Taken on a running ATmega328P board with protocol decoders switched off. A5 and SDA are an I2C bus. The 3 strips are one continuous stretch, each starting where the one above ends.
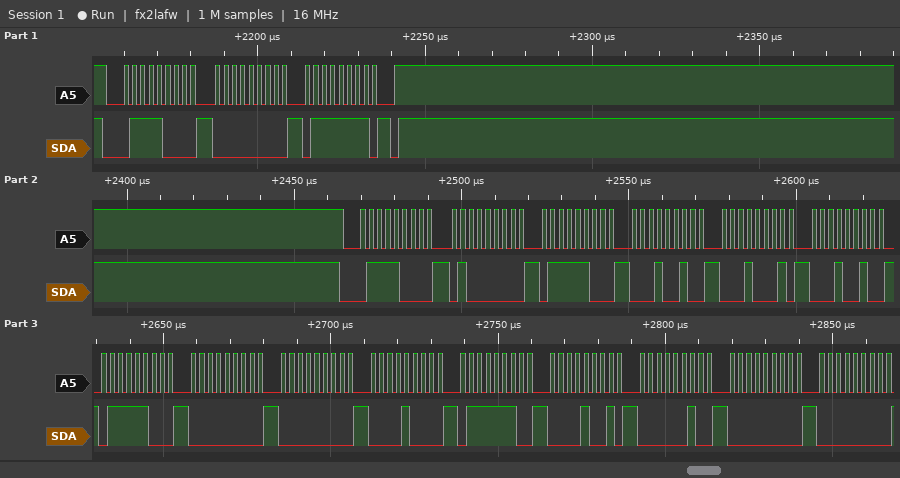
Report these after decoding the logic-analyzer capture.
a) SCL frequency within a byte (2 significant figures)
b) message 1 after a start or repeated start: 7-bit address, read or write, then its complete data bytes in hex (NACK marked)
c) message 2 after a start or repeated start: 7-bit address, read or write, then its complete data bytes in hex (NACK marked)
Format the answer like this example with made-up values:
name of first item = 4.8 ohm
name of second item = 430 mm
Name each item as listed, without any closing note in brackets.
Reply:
SCL frequency within a byte = 400 kHz
message 1 after a start or repeated start: 7-bit address, read or write, then its complete data bytes in hex = 0x3C write: 00 7F
message 2 after a start or repeated start: 7-bit address, read or write, then its complete data bytes in hex = 0x3C write: 40 7C 12 11 12 7C 00 00 08 7E 09 02 00 00
